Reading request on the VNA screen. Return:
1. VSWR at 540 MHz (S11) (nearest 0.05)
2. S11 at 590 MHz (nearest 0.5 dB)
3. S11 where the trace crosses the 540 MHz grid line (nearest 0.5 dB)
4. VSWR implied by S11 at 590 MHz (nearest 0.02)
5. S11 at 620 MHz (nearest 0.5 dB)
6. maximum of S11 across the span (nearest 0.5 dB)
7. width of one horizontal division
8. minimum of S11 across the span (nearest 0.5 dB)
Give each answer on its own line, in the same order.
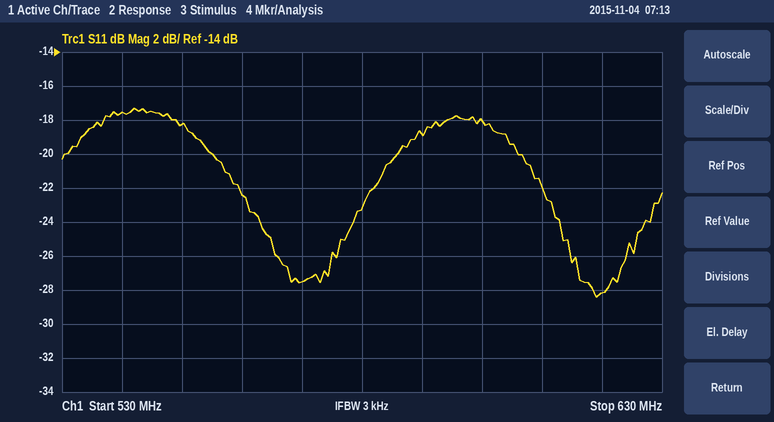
1.30
-19.0 dB
-17.5 dB
1.26
-28.0 dB
-17.5 dB
10 MHz
-28.5 dB
